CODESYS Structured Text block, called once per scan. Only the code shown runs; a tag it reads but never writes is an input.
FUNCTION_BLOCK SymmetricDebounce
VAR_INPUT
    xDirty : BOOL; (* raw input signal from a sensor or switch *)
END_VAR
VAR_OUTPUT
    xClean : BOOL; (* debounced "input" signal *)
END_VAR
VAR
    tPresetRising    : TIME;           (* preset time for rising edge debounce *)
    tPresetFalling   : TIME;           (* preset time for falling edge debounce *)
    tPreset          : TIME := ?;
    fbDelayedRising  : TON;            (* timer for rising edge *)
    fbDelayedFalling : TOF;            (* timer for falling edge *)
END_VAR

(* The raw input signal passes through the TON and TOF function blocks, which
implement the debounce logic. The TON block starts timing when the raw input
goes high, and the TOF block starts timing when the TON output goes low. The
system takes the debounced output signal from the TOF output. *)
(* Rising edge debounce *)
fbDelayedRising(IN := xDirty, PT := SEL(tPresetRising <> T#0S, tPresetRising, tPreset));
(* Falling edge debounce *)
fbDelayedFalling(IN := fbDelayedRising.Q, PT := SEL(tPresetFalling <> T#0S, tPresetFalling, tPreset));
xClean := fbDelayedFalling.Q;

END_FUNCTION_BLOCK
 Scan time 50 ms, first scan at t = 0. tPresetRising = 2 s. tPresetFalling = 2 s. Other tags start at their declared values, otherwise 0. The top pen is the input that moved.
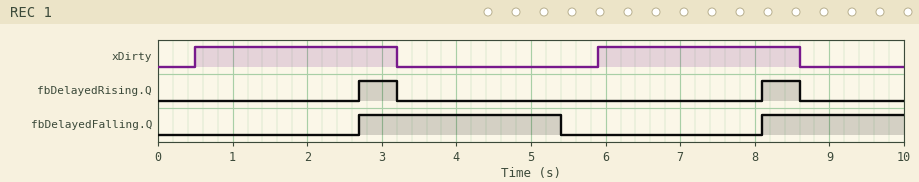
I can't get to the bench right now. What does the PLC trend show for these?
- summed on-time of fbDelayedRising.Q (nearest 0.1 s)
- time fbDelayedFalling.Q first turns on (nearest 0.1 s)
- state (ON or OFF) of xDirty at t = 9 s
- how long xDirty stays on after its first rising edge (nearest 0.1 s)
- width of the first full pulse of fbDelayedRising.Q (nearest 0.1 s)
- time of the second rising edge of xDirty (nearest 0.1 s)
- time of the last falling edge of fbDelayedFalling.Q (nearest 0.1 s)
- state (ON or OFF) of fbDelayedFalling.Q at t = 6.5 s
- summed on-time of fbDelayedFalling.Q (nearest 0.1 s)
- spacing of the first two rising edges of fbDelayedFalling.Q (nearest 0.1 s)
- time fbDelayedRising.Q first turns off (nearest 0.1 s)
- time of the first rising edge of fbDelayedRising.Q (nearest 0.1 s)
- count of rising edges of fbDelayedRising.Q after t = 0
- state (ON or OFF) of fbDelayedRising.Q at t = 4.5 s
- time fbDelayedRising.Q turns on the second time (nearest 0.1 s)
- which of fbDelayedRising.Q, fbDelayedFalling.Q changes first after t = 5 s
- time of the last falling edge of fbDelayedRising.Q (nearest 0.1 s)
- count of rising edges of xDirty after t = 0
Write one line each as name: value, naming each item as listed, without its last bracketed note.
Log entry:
summed on-time of fbDelayedRising.Q: 1.0 s
time fbDelayedFalling.Q first turns on: 2.7 s
state (ON or OFF) of xDirty at t = 9 s: OFF
how long xDirty stays on after its first rising edge: 2.7 s
width of the first full pulse of fbDelayedRising.Q: 0.5 s
time of the second rising edge of xDirty: 5.9 s
time of the last falling edge of fbDelayedFalling.Q: 5.4 s
state (ON or OFF) of fbDelayedFalling.Q at t = 6.5 s: OFF
summed on-time of fbDelayedFalling.Q: 4.6 s
spacing of the first two rising edges of fbDelayedFalling.Q: 5.4 s
time fbDelayedRising.Q first turns off: 3.2 s
time of the first rising edge of fbDelayedRising.Q: 2.7 s
count of rising edges of fbDelayedRising.Q after t = 0: 2
state (ON or OFF) of fbDelayedRising.Q at t = 4.5 s: OFF
time fbDelayedRising.Q turns on the second time: 8.1 s
which of fbDelayedRising.Q, fbDelayedFalling.Q changes first after t = 5 s: fbDelayedFalling.Q
time of the last falling edge of fbDelayedRising.Q: 8.6 s
count of rising edges of xDirty after t = 0: 2
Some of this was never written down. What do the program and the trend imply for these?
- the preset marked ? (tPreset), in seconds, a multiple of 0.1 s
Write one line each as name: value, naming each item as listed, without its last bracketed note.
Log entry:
the preset marked ? (tPreset), in seconds, a multiple of 0.1 s: 2.2 s
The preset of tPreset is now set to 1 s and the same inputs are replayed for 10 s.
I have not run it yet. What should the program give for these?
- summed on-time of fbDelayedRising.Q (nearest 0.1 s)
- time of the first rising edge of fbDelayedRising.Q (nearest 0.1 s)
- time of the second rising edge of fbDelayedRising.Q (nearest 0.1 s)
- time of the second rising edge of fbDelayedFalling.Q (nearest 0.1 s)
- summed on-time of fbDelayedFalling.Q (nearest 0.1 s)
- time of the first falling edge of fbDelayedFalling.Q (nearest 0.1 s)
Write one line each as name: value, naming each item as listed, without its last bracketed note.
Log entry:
summed on-time of fbDelayedRising.Q: 3.4 s
time of the first rising edge of fbDelayedRising.Q: 1.5 s
time of the second rising edge of fbDelayedRising.Q: 6.9 s
time of the second rising edge of fbDelayedFalling.Q: 6.9 s
summed on-time of fbDelayedFalling.Q: 5.4 s
time of the first falling edge of fbDelayedFalling.Q: 4.2 s
